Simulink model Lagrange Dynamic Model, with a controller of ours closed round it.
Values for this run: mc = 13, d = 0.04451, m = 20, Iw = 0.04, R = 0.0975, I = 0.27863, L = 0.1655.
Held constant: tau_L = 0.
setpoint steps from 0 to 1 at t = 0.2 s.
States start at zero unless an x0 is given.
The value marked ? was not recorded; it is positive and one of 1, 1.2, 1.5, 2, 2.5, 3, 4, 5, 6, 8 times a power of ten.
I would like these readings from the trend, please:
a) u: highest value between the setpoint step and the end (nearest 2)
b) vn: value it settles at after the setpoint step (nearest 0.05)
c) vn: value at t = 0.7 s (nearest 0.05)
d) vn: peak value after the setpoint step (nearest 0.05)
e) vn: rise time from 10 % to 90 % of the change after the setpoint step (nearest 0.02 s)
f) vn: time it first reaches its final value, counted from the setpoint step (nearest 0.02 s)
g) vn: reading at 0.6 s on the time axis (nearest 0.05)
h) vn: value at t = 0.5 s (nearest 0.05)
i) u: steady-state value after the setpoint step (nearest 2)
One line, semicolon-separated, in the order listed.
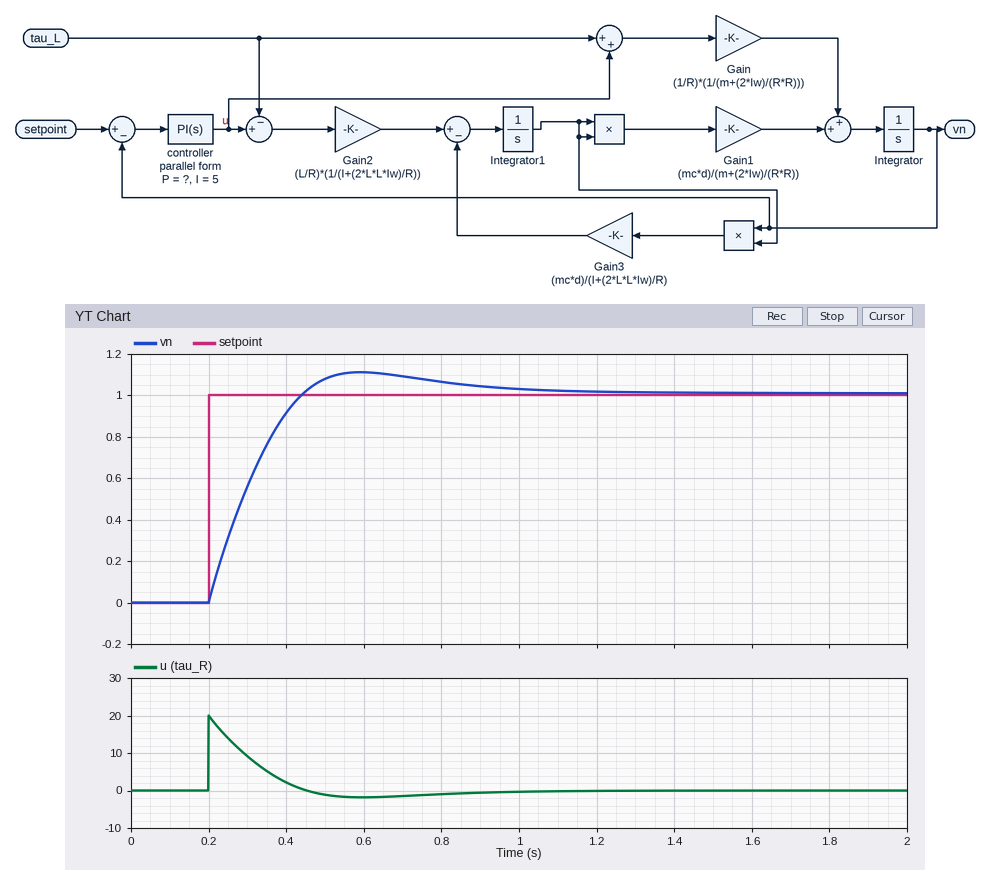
20; 1.00; 1.10; 1.10; 0.18 s; 0.24 s; 1.10; 1.10; 0
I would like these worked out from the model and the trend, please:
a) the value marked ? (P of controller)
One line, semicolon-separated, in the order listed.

20
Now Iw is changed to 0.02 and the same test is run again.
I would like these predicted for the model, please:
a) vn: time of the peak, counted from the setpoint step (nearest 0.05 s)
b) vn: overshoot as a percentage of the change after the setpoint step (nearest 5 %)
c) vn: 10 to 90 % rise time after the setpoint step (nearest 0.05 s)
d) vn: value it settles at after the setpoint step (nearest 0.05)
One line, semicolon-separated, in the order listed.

0.35 s; 10 %; 0.15 s; 1.00
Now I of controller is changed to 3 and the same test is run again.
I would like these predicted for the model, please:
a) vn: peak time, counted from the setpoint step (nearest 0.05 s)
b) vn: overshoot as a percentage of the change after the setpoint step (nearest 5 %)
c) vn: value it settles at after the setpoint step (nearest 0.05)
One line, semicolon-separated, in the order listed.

0.40 s; 10 %; 1.00
